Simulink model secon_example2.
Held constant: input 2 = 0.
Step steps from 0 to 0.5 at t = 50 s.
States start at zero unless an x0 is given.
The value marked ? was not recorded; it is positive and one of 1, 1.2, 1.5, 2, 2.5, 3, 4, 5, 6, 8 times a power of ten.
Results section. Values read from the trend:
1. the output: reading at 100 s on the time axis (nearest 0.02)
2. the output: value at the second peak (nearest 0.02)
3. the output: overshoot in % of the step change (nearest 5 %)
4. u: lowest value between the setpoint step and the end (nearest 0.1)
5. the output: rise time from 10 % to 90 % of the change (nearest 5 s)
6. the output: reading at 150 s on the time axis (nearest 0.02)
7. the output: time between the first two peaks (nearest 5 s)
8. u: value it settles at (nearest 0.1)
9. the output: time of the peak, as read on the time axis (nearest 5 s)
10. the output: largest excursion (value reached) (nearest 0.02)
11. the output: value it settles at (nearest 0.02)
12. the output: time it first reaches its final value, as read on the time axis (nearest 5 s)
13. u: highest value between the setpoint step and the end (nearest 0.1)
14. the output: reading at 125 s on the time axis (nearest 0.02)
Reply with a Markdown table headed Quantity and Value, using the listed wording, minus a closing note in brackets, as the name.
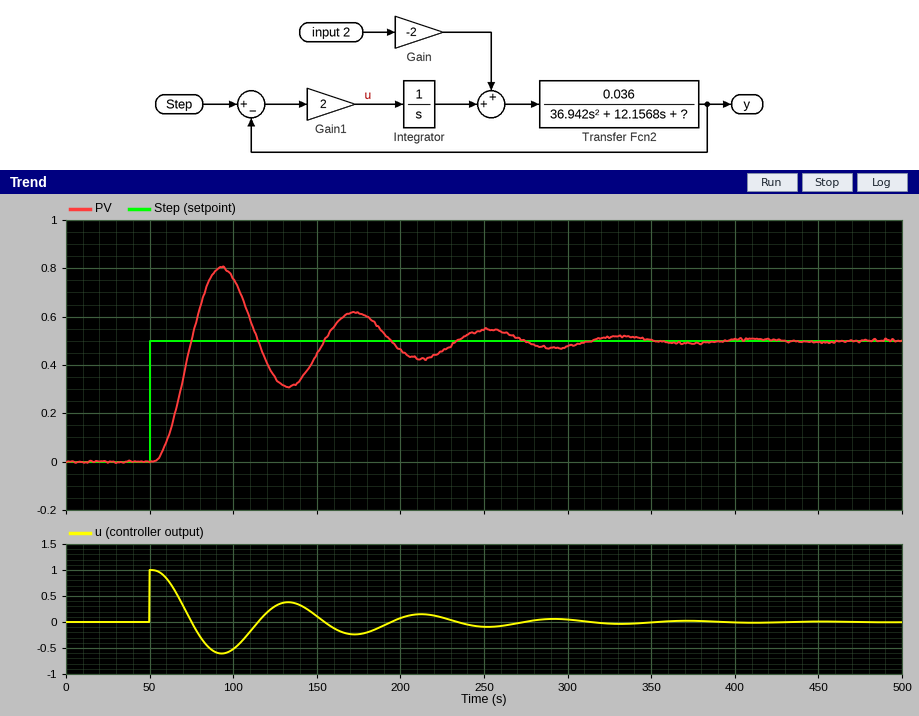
| Quantity | Value |
|---|---|
| the output: reading at 100 s on the time axis | 0.76 |
| the output: value at the second peak | 0.62 |
| the output: overshoot in % of the step change | 60 % |
| u: lowest value between the setpoint step and the end | -0.6 |
| the output: rise time from 10 % to 90 % of the change | 15 s |
| the output: reading at 150 s on the time axis | 0.44 |
| the output: time between the first two peaks | 80 s |
| u: value it settles at | 0.0 |
| the output: time of the peak, as read on the time axis | 95 s |
| the output: largest excursion (value reached) | 0.80 |
| the output: value it settles at | 0.50 |
| the output: time it first reaches its final value, as read on the time axis | 75 s |
| u: highest value between the setpoint step and the end | 1.0 |
| the output: reading at 125 s on the time axis | 0.34 |
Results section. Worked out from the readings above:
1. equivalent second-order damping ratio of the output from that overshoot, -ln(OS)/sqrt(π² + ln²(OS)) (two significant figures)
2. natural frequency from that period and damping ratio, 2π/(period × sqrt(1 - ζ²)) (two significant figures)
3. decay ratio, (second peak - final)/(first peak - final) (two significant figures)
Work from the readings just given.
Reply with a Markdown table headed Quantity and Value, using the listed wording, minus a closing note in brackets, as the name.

| Quantity | Value |
|---|---|
| equivalent second-order damping ratio of the output from that overshoot, -ln(OS)/sqrt(π² + ln²(OS)) | 0.16 |
| natural frequency from that period and damping ratio, 2π/(period × sqrt(1 - ζ²)) | 0.080 rad/s |
| decay ratio, (second peak - final)/(first peak - final) | 0.40 |
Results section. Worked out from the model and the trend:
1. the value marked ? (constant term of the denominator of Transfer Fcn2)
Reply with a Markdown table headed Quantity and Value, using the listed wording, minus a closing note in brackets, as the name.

| Quantity | Value |
|---|---|
| the value marked ? | 0.5 |
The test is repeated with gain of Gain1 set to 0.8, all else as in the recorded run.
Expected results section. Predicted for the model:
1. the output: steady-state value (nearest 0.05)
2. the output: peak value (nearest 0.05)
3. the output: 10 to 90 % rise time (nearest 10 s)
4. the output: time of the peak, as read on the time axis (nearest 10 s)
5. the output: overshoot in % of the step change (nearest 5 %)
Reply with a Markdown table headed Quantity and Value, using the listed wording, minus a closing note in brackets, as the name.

| Quantity | Value |
|---|---|
| the output: steady-state value | 0.50 |
| the output: peak value | 0.65 |
| the output: 10 to 90 % rise time | 30 s |
| the output: time of the peak, as read on the time axis | 120 s |
| the output: overshoot in % of the step change | 30 % |
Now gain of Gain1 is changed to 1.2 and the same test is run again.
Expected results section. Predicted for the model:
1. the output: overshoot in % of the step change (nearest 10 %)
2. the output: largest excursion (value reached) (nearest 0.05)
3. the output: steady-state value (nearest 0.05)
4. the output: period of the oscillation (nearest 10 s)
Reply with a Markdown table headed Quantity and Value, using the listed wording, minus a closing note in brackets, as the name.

| Quantity | Value |
|---|---|
| the output: overshoot in % of the step change | 40 % |
| the output: largest excursion (value reached) | 0.70 |
| the output: steady-state value | 0.50 |
| the output: period of the oscillation | 100 s |
